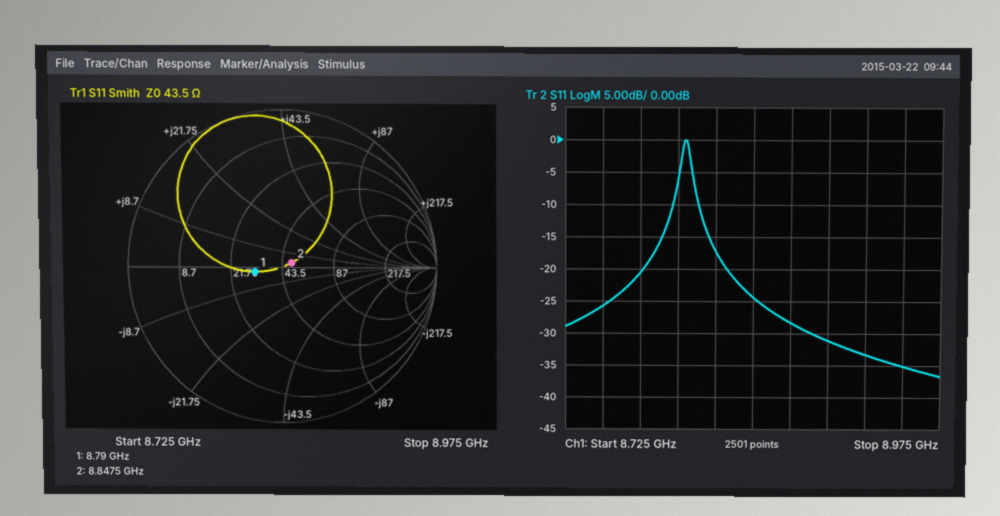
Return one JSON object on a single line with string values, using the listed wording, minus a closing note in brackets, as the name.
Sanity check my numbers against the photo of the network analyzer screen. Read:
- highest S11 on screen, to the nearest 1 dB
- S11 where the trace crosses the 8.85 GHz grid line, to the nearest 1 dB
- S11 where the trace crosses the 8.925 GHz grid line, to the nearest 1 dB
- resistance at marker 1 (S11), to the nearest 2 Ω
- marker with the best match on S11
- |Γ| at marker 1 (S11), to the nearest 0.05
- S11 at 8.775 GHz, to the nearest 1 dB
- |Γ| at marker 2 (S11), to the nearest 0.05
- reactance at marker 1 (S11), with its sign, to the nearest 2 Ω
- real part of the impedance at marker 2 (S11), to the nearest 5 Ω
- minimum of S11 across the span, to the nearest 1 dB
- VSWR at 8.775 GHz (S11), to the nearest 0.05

{"highest S11 on screen, to the nearest 1 dB": "0 dB", "S11 where the trace crosses the 8.85 GHz grid line, to the nearest 1 dB": "-24 dB", "S11 where the trace crosses the 8.925 GHz grid line, to the nearest 1 dB": "-33 dB", "resistance at marker 1 (S11), to the nearest 2 Ω": "30 Ω", "marker with the best match on S11": "marker 2", "|Γ| at marker 1 (S11), to the nearest 0.05": "0.20", "S11 at 8.775 GHz, to the nearest 1 dB": "-21 dB", "|Γ| at marker 2 (S11), to the nearest 0.05": "0.05", "reactance at marker 1 (S11), with its sign, to the nearest 2 Ω": "-2 Ω", "real part of the impedance at marker 2 (S11), to the nearest 5 Ω": "50 Ω", "minimum of S11 across the span, to the nearest 1 dB": "-37 dB", "VSWR at 8.775 GHz (S11), to the nearest 0.05": "1.20"}
